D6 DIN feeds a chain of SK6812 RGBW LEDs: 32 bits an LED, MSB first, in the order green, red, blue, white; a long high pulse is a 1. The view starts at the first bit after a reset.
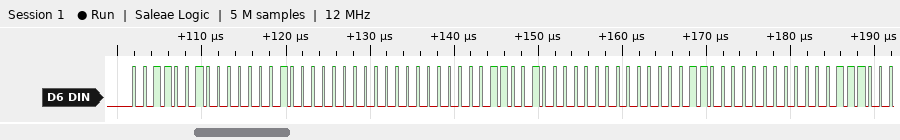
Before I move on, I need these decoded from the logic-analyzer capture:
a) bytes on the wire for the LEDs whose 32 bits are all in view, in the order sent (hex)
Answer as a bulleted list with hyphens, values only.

- 32 02 00 00 32 00 06 00
